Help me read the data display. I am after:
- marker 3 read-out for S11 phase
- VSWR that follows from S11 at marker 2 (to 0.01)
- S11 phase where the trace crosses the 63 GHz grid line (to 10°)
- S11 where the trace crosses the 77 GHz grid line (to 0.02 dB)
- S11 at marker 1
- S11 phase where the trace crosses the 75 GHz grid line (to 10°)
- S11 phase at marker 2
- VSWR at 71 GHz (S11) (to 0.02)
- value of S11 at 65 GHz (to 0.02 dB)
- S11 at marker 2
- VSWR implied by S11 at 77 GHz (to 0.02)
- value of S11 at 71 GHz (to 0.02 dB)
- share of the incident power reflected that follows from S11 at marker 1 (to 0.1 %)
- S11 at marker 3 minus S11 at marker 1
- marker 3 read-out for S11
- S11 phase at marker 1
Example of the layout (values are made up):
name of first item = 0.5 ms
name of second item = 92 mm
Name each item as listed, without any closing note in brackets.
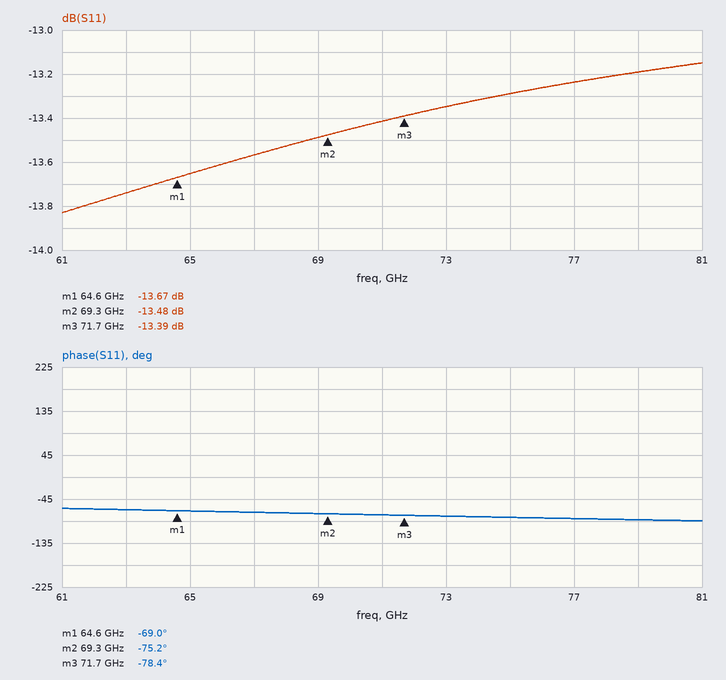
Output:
marker 3 read-out for S11 phase = -78.4°
VSWR that follows from S11 at marker 2 = 1.54
S11 phase where the trace crosses the 63 GHz grid line = -70°
S11 where the trace crosses the 77 GHz grid line = -13.24 dB
S11 at marker 1 = -13.67 dB
S11 phase where the trace crosses the 75 GHz grid line = -80°
S11 phase at marker 2 = -75.2°
VSWR at 71 GHz (S11) = 1.54
value of S11 at 65 GHz = -13.66 dB
S11 at marker 2 = -13.48 dB
VSWR implied by S11 at 77 GHz = 1.56
value of S11 at 71 GHz = -13.42 dB
share of the incident power reflected that follows from S11 at marker 1 = 4.3 %
S11 at marker 3 minus S11 at marker 1 = 0.28 dB
marker 3 read-out for S11 = -13.39 dB
S11 phase at marker 1 = -69.0°
